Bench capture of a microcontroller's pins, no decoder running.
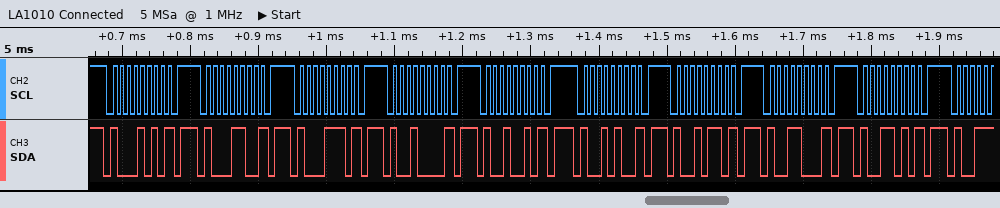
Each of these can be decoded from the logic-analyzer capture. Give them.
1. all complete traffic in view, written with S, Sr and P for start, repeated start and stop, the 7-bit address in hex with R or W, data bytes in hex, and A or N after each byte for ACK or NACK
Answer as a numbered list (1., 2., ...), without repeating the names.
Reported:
1. S 45W N P S 46W N P S 47W N P S 48W N P S 49W N P S 4AW N P S 4BW N P S 4CW N P S 4DW N P
